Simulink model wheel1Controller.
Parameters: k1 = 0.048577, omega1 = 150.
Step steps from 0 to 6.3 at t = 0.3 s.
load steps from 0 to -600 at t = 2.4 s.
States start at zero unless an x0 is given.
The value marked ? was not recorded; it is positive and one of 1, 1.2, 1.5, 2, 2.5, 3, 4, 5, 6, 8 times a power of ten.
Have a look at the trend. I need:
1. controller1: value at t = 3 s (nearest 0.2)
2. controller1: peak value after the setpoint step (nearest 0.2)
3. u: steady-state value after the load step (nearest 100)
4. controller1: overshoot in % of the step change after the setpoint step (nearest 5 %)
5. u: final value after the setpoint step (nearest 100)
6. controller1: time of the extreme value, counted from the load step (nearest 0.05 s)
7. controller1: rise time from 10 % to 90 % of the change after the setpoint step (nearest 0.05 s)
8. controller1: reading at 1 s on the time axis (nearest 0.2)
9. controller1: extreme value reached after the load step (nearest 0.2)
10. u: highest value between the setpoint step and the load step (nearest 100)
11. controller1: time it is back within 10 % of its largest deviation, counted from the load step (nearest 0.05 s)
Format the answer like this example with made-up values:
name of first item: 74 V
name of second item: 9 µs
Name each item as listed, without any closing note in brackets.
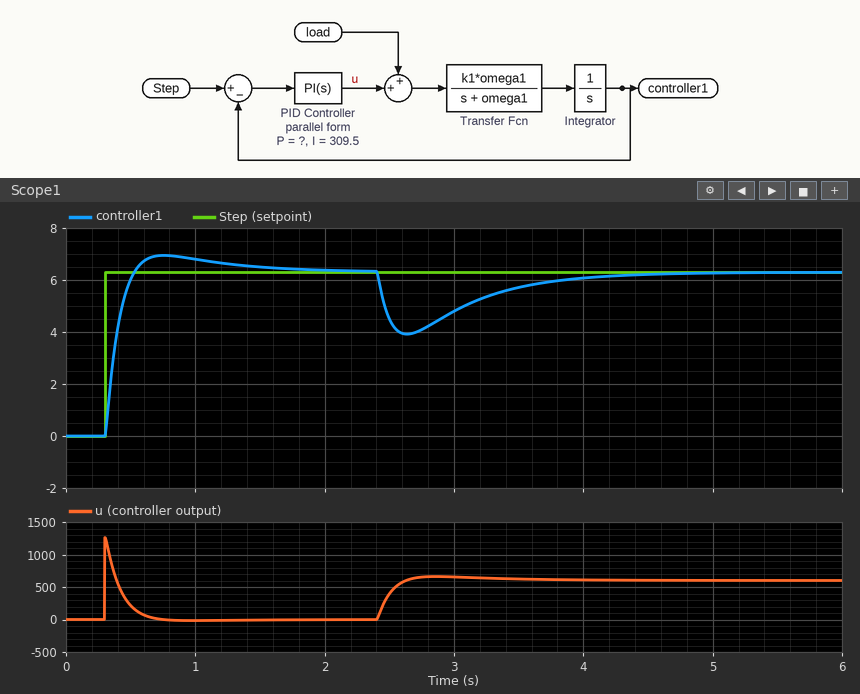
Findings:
controller1: value at t = 3 s: 4.8
controller1: peak value after the setpoint step: 7.0
u: steady-state value after the load step: 600
controller1: overshoot in % of the step change after the setpoint step: 10 %
u: final value after the setpoint step: 0
controller1: time of the extreme value, counted from the load step: 0.25 s
controller1: rise time from 10 % to 90 % of the change after the setpoint step: 0.15 s
controller1: reading at 1 s on the time axis: 6.8
controller1: extreme value reached after the load step: 4.0
u: highest value between the setpoint step and the load step: 1300
controller1: time it is back within 10 % of its largest deviation, counted from the load step: 1.55 s
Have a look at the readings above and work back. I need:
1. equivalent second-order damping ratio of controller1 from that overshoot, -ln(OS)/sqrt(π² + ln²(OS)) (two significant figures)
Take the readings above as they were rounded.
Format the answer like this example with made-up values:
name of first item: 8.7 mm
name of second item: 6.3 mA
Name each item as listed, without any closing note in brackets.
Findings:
equivalent second-order damping ratio of controller1 from that overshoot, -ln(OS)/sqrt(π² + ln²(OS)): 0.59
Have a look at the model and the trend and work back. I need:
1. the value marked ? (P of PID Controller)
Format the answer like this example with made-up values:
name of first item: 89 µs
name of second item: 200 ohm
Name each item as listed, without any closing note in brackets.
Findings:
the value marked ?: 200
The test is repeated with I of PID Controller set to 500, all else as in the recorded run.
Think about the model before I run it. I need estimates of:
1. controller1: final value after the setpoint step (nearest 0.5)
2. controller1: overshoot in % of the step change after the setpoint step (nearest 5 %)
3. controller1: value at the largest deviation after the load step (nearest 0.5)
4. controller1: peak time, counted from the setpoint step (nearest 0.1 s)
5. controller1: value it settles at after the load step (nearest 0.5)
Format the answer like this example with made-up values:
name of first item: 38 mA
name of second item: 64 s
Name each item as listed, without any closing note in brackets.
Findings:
controller1: final value after the setpoint step: 6.5
controller1: overshoot in % of the step change after the setpoint step: 15 %
controller1: value at the largest deviation after the load step: 4.0
controller1: peak time, counted from the setpoint step: 0.4 s
controller1: value it settles at after the load step: 6.5
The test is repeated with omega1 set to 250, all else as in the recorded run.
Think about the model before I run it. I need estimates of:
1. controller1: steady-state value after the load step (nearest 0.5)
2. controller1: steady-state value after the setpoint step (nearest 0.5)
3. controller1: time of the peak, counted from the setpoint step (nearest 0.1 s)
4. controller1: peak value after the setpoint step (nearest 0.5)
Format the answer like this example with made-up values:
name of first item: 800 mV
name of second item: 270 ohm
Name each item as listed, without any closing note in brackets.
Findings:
controller1: steady-state value after the load step: 6.5
controller1: steady-state value after the setpoint step: 6.5
controller1: time of the peak, counted from the setpoint step: 0.5 s
controller1: peak value after the setpoint step: 7.0
